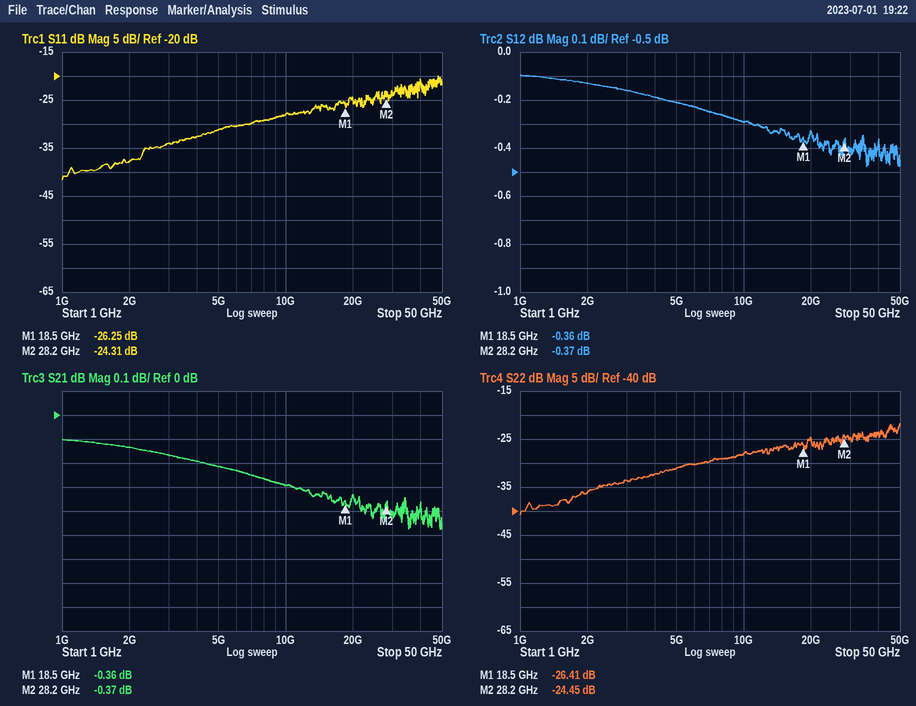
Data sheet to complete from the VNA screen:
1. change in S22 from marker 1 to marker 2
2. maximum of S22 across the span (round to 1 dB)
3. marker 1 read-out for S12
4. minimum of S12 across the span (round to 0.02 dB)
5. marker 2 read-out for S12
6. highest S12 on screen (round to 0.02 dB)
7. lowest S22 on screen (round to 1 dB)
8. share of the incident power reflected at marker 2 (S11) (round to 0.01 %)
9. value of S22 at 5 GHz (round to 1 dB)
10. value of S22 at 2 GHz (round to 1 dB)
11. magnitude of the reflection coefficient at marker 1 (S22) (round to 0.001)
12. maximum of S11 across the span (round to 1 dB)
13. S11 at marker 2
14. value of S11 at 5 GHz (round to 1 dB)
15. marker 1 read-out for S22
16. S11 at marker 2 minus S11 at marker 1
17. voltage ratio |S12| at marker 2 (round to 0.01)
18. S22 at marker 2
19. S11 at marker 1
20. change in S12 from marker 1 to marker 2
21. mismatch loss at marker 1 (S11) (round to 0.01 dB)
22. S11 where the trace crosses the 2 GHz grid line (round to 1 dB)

1.96 dB
-22 dB
-0.36 dB
-0.48 dB
-0.37 dB
-0.10 dB
-41 dB
0.37 %
-31 dB
-36 dB
0.048
-20 dB
-24.31 dB
-31 dB
-26.41 dB
1.94 dB
0.96
-24.45 dB
-26.25 dB
-0.01 dB
0.01 dB
-38 dB
